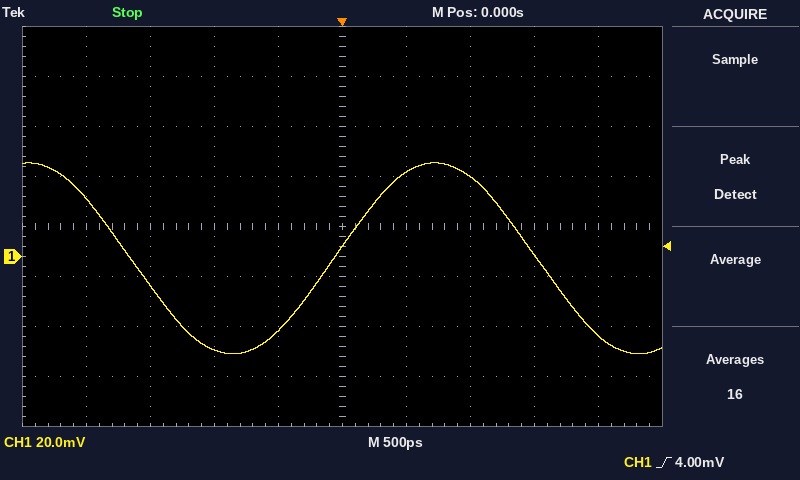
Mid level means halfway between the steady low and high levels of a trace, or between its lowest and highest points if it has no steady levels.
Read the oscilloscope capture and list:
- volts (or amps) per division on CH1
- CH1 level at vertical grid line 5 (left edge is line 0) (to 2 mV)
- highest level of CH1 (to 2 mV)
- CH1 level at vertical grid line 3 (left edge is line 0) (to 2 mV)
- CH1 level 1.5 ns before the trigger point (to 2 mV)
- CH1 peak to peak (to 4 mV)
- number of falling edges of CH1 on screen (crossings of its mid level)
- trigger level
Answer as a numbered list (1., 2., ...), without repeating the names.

1. 20 mV
2. 4 mV
3. 38 mV
4. -38 mV
5. -12 mV
6. 76 mV
7. 2
8. 4.00 mV
